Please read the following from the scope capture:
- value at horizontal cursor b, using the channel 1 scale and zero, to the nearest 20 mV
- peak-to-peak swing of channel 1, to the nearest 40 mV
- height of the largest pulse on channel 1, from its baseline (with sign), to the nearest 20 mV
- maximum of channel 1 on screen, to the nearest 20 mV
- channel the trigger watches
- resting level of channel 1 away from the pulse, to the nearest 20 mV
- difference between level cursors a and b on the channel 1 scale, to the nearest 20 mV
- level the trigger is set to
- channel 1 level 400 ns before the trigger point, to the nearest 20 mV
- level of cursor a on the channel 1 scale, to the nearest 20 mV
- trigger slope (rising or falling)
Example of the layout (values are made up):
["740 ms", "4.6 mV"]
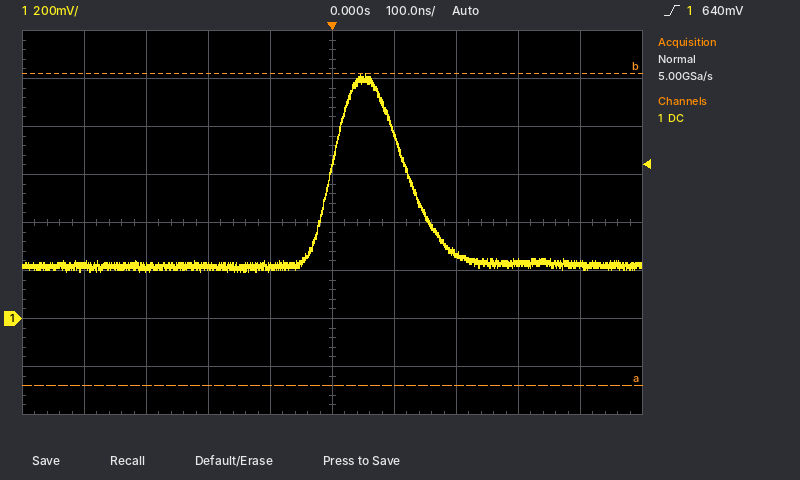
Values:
["1.02 V", "840 mV", "+800 mV", "1.02 V", "channel 1", "220 mV", "1.30 V", "640 mV", "220 mV", "-280 mV", "rising"]
